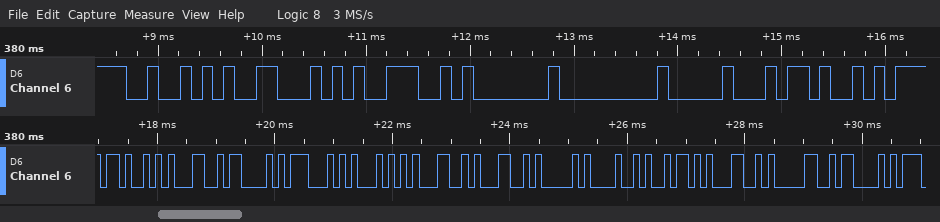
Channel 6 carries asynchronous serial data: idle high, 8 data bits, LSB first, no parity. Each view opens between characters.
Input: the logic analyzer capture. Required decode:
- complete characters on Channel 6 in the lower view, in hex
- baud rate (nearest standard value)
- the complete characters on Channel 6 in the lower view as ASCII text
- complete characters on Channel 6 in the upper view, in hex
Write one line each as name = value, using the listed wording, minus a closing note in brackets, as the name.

complete characters on Channel 6 in the lower view, in hex = 4B, 31, 43, 47, 51, 31, 31, 41, 48, 5A, 4C, 30, 43
baud rate = 9600 baud
the complete characters on Channel 6 in the lower view as ASCII text = "K1CGQ11AHZL0C"
complete characters on Channel 6 in the upper view, in hex = 52, 46, 39, 01, 00, 10, 4B
